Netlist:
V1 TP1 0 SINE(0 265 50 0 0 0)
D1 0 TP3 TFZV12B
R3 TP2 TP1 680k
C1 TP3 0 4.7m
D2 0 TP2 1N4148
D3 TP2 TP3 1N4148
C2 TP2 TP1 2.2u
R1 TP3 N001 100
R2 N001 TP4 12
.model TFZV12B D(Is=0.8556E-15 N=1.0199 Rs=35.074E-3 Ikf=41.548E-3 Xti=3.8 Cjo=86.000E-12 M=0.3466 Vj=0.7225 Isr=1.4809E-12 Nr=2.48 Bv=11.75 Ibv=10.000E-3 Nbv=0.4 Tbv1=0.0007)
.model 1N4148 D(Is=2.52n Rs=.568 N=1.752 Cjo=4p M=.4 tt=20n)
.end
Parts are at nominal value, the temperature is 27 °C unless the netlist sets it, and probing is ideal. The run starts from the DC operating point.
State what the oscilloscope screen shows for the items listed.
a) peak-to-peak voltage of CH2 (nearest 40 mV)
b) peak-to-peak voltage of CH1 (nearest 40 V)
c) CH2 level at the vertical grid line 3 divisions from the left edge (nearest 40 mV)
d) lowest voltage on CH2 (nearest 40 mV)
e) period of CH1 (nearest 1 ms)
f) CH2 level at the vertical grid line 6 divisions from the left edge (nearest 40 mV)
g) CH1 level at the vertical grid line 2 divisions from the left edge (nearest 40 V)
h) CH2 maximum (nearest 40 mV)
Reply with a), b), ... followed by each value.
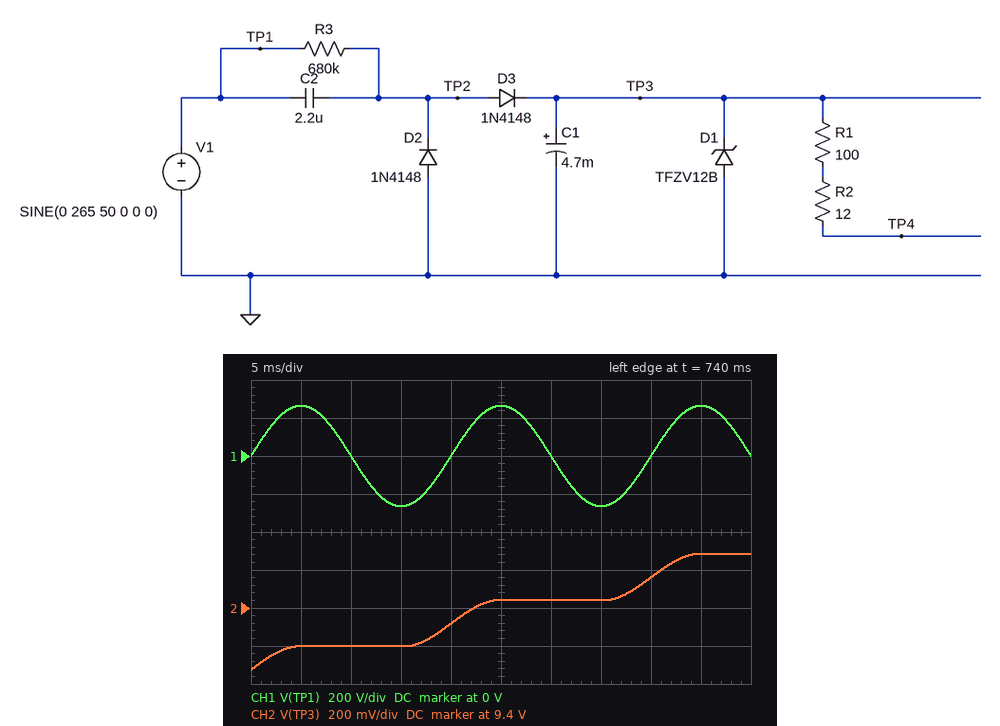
a) 600 mV
b) 520 V
c) 9.20 V
d) 9.08 V
e) 20 ms
f) 9.44 V
g) 0 V
h) 9.68 V
